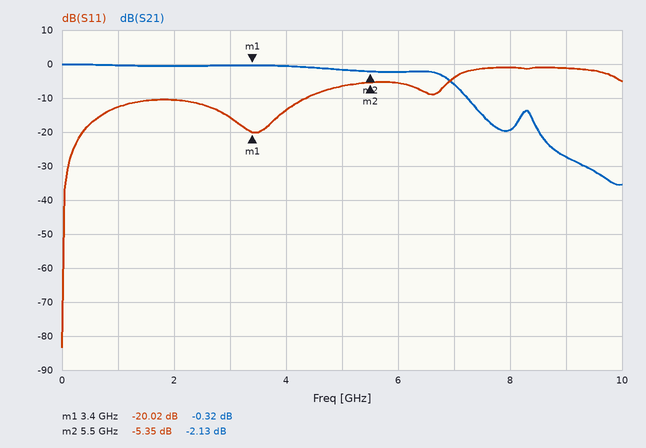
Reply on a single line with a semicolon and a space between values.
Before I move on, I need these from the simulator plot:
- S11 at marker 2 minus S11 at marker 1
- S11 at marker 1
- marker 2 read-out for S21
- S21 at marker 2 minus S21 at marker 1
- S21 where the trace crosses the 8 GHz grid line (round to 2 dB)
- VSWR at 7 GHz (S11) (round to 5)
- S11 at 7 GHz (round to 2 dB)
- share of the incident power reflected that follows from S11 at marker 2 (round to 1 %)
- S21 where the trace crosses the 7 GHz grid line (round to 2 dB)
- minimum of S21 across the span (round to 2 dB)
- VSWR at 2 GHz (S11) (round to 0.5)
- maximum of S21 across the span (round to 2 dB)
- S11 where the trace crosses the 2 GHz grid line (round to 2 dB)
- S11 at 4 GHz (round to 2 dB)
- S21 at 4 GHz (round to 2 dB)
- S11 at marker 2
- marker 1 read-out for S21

14.67 dB; -20.02 dB; -2.13 dB; -1.81 dB; -20 dB; 5; -4 dB; 29 %; -6 dB; -36 dB; 2.0; 0 dB; -10 dB; -14 dB; 0 dB; -5.35 dB; -0.32 dB
